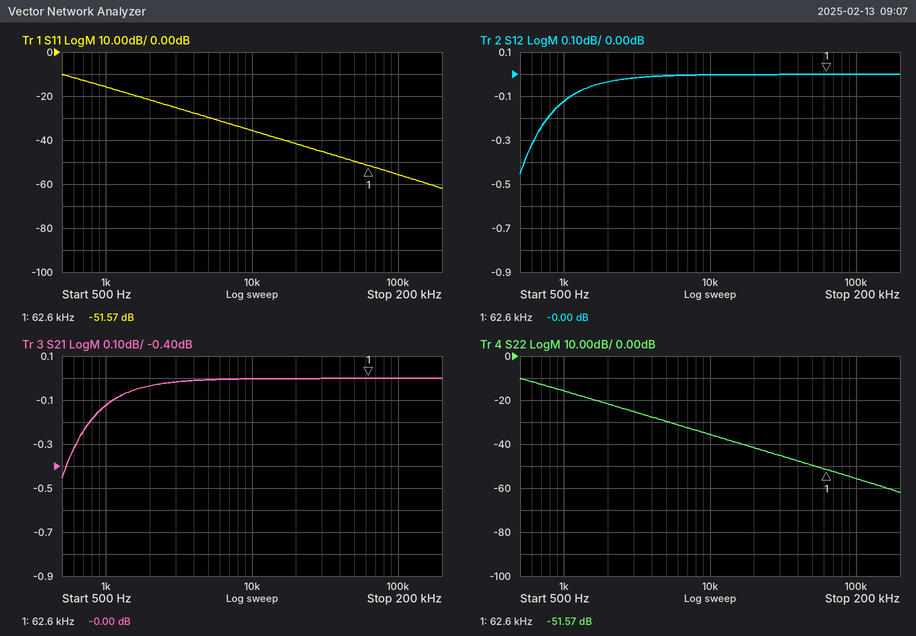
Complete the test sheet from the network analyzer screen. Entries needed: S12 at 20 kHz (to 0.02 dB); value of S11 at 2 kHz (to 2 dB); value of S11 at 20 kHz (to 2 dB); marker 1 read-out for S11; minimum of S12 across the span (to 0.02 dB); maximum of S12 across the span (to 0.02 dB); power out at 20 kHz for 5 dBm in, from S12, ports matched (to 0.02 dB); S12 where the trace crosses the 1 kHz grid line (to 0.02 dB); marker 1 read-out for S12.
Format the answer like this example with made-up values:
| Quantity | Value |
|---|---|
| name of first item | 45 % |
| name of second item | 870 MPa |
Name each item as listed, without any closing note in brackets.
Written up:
| Quantity | Value |
|---|---|
| S12 at 20 kHz | 0.00 dB |
| value of S11 at 2 kHz | -22 dB |
| value of S11 at 20 kHz | -42 dB |
| marker 1 read-out for S11 | -51.57 dB |
| minimum of S12 across the span | -0.46 dB |
| maximum of S12 across the span | 0.00 dB |
| power out at 20 kHz for 5 dBm in, from S12, ports matched | 5.00 dBm |
| S12 where the trace crosses the 1 kHz grid line | -0.12 dB |
| marker 1 read-out for S12 | -0.00 dB |
